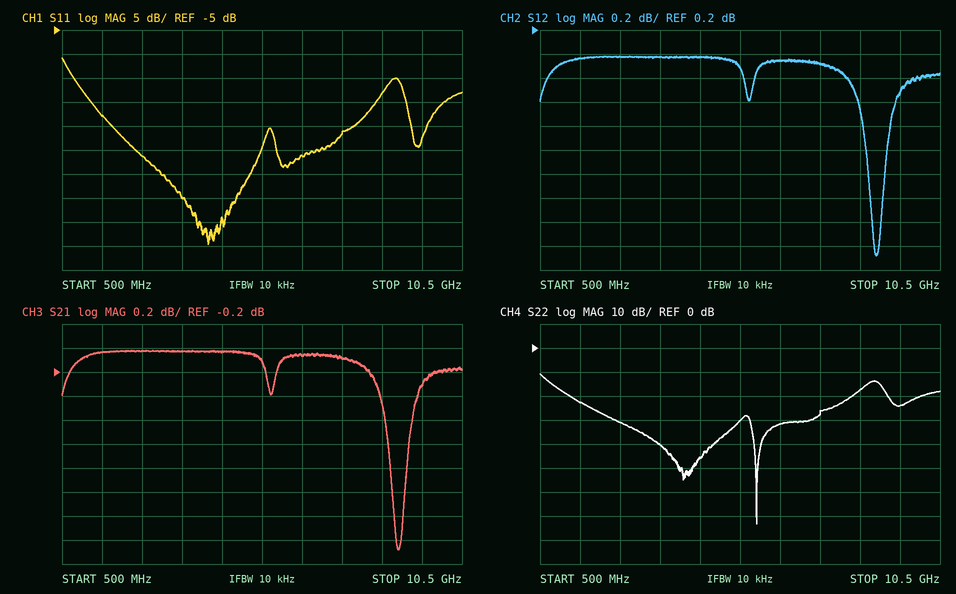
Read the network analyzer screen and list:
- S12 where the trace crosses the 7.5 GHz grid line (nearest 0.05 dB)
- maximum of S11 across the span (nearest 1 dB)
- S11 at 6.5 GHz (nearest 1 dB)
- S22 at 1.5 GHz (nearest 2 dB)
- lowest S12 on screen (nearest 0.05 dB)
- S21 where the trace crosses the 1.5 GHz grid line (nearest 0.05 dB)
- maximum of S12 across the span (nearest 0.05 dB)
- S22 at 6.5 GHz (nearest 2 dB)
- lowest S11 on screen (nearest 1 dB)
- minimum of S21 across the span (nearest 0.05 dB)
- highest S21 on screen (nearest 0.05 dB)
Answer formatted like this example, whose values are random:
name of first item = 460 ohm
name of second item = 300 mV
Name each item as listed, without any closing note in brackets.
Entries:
S12 where the trace crosses the 7.5 GHz grid line = -0.10 dB
maximum of S11 across the span = -11 dB
S11 at 6.5 GHz = -31 dB
S22 at 1.5 GHz = -22 dB
lowest S12 on screen = -1.70 dB
S21 where the trace crosses the 1.5 GHz grid line = -0.05 dB
maximum of S12 across the span = 0.00 dB
S22 at 6.5 GHz = -32 dB
lowest S11 on screen = -50 dB
minimum of S21 across the span = -1.70 dB
highest S21 on screen = 0.00 dB
